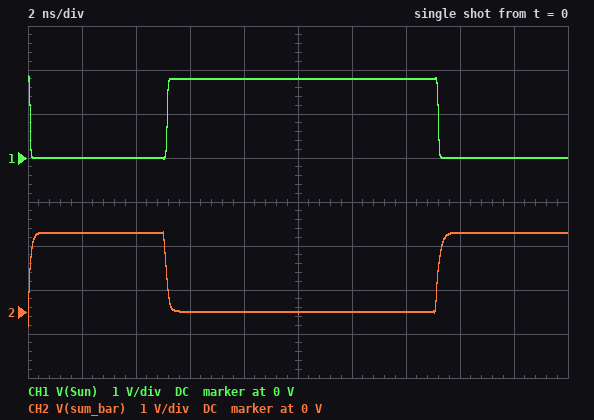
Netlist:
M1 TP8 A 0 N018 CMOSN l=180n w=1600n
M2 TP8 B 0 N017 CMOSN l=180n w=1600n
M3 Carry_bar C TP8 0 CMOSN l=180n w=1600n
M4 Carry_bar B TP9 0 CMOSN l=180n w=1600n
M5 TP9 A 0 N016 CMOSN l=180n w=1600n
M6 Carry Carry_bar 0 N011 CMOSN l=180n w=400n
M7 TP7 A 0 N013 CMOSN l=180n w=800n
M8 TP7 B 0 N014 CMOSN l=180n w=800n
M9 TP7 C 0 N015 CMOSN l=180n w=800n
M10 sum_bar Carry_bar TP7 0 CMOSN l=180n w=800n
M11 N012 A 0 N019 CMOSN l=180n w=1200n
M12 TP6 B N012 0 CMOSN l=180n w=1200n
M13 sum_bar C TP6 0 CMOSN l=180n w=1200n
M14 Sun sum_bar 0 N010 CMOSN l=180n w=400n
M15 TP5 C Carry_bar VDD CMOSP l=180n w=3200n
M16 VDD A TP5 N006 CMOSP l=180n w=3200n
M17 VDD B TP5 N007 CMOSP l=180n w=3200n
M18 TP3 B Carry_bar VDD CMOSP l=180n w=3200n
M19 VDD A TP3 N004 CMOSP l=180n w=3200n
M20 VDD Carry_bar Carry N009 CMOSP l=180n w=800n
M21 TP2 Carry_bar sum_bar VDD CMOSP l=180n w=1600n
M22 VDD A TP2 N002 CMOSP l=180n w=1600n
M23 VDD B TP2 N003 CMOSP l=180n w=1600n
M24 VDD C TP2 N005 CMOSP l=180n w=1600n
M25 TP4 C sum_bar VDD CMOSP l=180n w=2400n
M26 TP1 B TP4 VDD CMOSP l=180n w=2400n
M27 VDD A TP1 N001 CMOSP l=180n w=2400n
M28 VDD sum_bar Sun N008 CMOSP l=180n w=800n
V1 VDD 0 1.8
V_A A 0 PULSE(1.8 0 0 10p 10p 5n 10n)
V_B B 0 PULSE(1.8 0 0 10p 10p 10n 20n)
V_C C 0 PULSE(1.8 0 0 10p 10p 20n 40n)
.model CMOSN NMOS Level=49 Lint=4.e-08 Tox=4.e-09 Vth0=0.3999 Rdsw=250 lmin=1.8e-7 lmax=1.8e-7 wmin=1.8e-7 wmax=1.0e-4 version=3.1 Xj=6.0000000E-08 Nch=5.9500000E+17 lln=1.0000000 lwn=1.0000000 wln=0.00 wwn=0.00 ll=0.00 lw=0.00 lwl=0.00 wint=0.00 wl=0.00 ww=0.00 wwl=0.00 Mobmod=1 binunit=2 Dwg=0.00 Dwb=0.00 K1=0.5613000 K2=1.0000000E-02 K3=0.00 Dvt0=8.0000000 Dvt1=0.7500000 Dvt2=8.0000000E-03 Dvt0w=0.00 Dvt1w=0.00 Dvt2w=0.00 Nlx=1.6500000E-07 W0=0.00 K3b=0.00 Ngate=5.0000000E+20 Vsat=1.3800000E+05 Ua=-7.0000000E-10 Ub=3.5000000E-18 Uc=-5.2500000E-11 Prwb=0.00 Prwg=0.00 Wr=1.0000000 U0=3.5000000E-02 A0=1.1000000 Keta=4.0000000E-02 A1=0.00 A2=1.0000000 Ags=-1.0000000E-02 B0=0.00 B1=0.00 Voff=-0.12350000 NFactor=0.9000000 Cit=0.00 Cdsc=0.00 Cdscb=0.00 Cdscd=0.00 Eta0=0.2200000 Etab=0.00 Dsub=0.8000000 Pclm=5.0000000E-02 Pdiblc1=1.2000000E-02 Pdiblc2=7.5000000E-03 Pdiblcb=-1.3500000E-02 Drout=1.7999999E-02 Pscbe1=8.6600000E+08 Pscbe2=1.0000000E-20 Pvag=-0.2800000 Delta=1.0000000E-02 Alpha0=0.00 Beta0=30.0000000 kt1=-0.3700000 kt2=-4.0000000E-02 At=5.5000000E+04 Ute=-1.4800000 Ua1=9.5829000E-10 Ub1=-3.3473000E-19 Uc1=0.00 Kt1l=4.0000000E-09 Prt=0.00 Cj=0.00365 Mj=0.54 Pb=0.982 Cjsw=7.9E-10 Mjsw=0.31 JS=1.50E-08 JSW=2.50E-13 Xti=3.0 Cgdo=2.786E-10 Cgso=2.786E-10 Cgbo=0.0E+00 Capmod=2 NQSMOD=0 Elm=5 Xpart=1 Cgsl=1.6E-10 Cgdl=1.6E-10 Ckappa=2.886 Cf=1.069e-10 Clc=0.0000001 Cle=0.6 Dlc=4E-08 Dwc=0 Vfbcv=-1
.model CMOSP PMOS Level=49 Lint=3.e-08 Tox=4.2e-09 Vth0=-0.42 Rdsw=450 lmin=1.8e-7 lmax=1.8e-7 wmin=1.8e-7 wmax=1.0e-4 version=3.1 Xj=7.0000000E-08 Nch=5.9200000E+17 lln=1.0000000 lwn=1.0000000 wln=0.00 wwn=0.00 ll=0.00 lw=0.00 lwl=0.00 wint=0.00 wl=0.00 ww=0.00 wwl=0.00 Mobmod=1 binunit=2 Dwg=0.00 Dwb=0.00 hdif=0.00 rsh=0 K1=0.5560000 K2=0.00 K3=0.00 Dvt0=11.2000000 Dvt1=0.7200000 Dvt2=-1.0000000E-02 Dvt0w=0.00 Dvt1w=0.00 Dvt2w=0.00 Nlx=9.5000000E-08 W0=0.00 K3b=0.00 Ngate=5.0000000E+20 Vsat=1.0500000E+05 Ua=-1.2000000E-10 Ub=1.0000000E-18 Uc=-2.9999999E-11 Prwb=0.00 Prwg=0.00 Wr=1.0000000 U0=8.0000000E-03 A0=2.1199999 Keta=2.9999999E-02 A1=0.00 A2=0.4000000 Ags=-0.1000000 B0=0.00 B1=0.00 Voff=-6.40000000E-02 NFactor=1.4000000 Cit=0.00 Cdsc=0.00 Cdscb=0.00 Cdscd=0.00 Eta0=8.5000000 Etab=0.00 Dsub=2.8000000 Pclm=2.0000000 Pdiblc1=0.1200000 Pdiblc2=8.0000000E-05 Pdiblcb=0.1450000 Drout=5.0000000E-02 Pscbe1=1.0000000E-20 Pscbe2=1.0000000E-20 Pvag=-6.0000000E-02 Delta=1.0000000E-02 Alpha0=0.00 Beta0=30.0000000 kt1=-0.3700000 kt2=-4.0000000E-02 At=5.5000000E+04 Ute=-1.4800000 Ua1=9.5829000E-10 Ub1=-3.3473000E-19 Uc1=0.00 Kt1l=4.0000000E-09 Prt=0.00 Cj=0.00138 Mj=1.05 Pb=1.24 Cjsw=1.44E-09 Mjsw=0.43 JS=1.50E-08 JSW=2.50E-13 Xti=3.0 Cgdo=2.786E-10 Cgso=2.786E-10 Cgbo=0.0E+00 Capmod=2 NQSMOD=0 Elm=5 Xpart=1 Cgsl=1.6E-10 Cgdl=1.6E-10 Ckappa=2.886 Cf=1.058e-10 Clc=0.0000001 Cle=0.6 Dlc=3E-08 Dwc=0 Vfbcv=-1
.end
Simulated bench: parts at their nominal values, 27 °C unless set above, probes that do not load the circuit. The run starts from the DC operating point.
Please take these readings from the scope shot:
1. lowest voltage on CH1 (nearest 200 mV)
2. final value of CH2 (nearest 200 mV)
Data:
0 V
1.8 V
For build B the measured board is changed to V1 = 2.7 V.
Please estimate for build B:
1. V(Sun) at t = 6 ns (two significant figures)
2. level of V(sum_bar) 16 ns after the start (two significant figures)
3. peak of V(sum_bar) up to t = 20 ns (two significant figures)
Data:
2.6 V
1.6 V
2.7 V
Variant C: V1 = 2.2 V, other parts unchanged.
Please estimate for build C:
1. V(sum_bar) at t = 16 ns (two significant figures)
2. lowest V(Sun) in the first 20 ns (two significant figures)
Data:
2.2 V
-19 mV
